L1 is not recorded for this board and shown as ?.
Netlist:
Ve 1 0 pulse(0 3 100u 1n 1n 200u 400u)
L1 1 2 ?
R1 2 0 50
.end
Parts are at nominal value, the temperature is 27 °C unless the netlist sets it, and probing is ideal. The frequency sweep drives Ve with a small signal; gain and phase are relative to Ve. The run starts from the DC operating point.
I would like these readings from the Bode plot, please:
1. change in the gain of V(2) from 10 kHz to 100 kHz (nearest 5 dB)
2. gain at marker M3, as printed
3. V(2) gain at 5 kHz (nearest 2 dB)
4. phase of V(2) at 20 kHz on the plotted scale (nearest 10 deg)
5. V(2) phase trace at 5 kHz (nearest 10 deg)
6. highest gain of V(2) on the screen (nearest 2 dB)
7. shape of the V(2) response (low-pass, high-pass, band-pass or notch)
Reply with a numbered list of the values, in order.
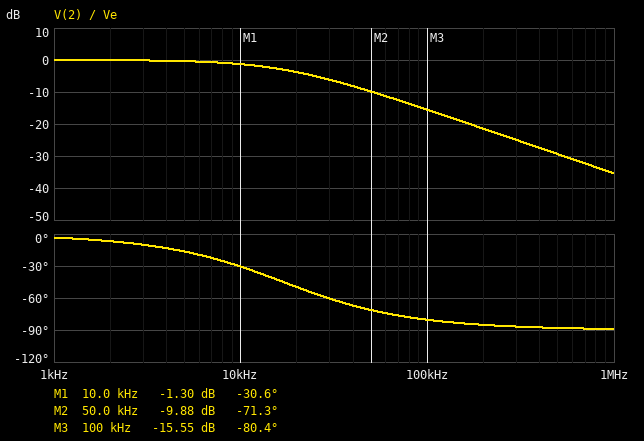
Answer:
1. -15 dB
2. -15.55 dB
3. 0 dB
4. -50 deg
5. -20 deg
6. 0 dB
7. low-pass
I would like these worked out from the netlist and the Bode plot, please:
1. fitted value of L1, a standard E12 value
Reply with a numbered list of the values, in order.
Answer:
1. 470 µH
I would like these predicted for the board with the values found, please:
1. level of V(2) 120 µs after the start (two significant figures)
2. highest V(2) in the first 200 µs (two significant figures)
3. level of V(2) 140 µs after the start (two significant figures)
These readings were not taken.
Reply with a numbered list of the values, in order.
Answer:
1. 2.6 V
2. 3.0 V
3. 3.0 V
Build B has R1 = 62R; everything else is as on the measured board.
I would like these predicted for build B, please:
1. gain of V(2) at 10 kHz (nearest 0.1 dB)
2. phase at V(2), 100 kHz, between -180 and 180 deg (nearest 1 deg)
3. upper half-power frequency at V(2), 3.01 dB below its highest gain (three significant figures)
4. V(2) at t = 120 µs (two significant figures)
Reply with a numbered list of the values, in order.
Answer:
1. -0.9 dB
2. -78 deg
3. 21.0 kHz
4. 2.8 V
